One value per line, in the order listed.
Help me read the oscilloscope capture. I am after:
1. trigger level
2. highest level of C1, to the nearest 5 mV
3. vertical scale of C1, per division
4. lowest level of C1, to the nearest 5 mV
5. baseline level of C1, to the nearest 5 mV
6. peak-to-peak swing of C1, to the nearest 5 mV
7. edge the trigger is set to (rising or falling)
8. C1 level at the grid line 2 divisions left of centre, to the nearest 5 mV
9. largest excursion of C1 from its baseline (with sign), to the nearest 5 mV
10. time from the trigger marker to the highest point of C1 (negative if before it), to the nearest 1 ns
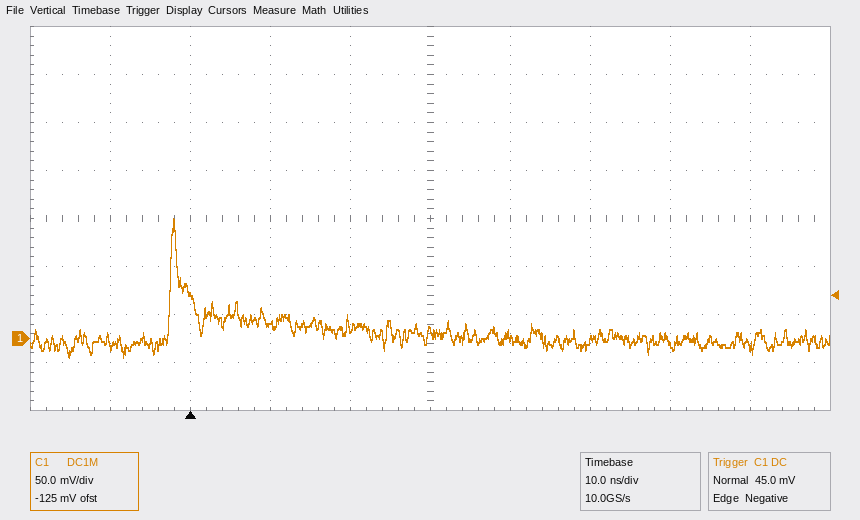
45.0 mV
125 mV
50 mV
-20 mV
0 mV
145 mV
falling
15 mV
+125 mV
-2 ns
